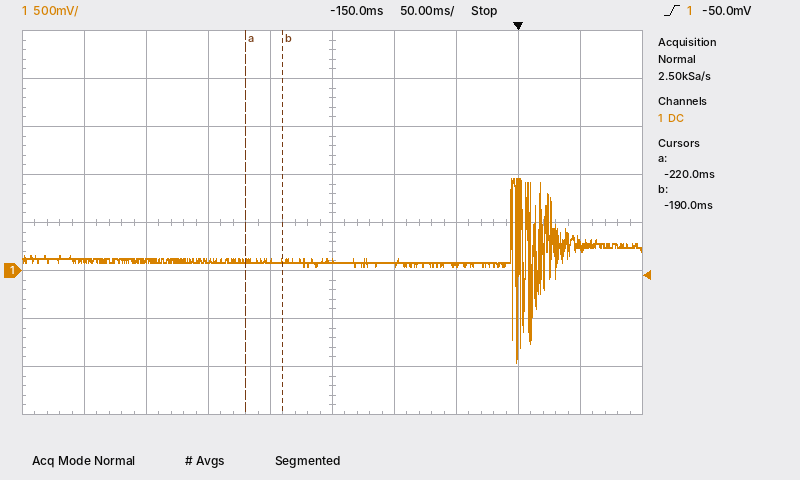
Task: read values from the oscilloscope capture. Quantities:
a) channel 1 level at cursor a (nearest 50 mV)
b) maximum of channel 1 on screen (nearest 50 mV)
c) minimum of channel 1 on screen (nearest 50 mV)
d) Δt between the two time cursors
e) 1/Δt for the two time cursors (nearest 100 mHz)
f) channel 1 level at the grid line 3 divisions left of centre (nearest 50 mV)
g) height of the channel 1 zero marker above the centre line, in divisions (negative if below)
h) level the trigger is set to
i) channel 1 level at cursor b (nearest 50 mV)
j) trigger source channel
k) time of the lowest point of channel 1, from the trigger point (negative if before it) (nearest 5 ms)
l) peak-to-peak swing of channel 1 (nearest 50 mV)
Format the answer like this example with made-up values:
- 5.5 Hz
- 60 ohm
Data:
- 100 mV
- 950 mV
- -950 mV
- 30 ms
- 33.3 Hz
- 100 mV
- -1.0 div
- -50.0 mV
- 100 mV
- channel 1
- 0 ms
- 1.90 V
